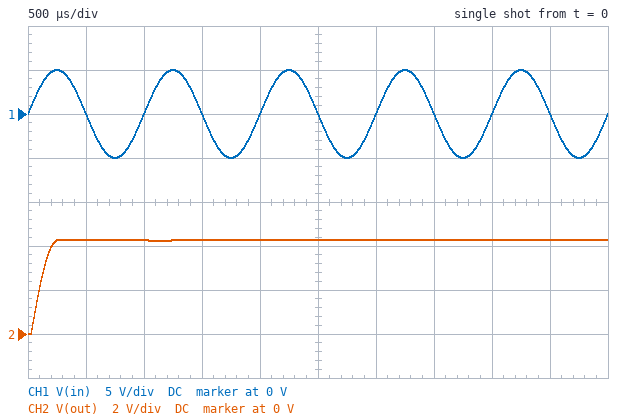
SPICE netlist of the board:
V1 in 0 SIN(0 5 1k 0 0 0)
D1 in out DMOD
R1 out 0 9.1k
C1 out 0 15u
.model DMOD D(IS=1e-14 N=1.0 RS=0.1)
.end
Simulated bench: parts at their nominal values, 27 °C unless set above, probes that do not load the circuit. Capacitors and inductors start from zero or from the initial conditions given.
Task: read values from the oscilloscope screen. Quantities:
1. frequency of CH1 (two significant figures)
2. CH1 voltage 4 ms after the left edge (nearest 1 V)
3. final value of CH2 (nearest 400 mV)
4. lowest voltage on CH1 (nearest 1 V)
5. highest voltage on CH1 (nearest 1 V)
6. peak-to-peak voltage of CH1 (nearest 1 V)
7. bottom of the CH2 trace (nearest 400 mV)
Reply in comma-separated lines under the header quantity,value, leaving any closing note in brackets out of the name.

quantity,value
frequency of CH1,1.0 kHz
CH1 voltage 4 ms after the left edge,0 V
final value of CH2,4.4 V
lowest voltage on CH1,-5 V
highest voltage on CH1,5 V
peak-to-peak voltage of CH1,10 V
bottom of the CH2 trace,0 V
